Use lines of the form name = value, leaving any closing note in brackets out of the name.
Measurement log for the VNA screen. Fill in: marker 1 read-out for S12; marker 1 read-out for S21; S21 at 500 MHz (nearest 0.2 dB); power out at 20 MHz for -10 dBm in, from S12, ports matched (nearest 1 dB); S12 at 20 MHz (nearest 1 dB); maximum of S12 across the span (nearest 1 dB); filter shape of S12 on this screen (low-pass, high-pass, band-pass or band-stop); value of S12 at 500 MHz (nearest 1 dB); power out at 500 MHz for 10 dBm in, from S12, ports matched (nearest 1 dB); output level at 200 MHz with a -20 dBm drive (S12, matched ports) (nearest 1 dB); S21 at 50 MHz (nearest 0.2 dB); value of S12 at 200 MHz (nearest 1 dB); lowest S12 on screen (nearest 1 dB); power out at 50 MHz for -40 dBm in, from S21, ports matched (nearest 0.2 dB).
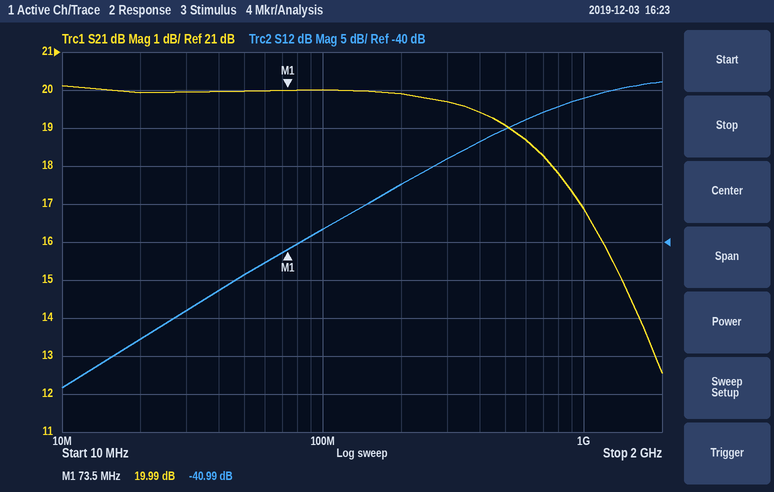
marker 1 read-out for S12 = -40.99 dB
marker 1 read-out for S21 = 19.99 dB
S21 at 500 MHz = 19.0 dB
power out at 20 MHz for -10 dBm in, from S12, ports matched = -63 dBm
S12 at 20 MHz = -53 dB
maximum of S12 across the span = -19 dB
filter shape of S12 on this screen = high-pass
value of S12 at 500 MHz = -25 dB
power out at 500 MHz for 10 dBm in, from S12, ports matched = -15 dBm
output level at 200 MHz with a -20 dBm drive (S12, matched ports) = -52 dBm
S21 at 50 MHz = 20.0 dB
value of S12 at 200 MHz = -32 dB
lowest S12 on screen = -59 dB
power out at 50 MHz for -40 dBm in, from S21, ports matched = -20.0 dBm
